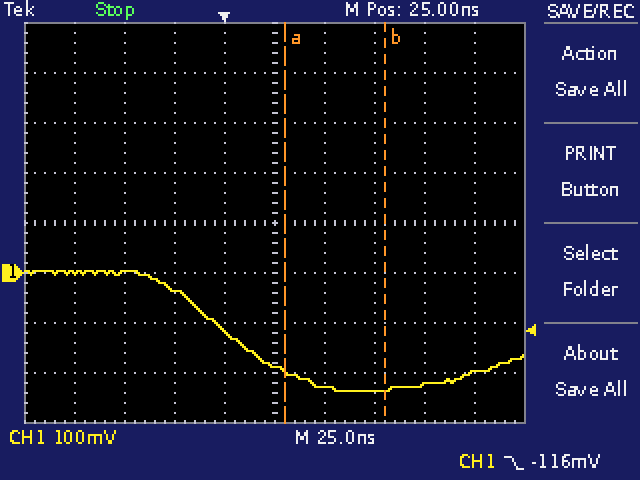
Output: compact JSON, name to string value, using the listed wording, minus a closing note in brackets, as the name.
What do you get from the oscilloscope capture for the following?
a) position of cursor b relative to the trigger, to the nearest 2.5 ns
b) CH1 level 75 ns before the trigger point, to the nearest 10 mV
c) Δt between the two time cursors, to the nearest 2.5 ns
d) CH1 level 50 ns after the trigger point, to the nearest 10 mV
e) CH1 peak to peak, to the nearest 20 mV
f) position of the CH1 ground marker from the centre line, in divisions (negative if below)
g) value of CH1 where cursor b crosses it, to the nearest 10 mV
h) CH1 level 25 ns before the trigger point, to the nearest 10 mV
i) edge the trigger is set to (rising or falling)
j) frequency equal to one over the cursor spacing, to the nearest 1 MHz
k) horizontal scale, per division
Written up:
{"position of cursor b relative to the trigger, to the nearest 2.5 ns": "+80.0 ns", "CH1 level 75 ns before the trigger point, to the nearest 10 mV": "0 mV", "Δt between the two time cursors, to the nearest 2.5 ns": "50.0 ns", "CH1 level 50 ns after the trigger point, to the nearest 10 mV": "-230 mV", "CH1 peak to peak, to the nearest 20 mV": "240 mV", "position of the CH1 ground marker from the centre line, in divisions": "-1.0 div", "value of CH1 where cursor b crosses it, to the nearest 10 mV": "-230 mV", "CH1 level 25 ns before the trigger point, to the nearest 10 mV": "-30 mV", "edge the trigger is set to": "falling", "frequency equal to one over the cursor spacing, to the nearest 1 MHz": "20 MHz", "horizontal scale, per division": "25 ns"}
